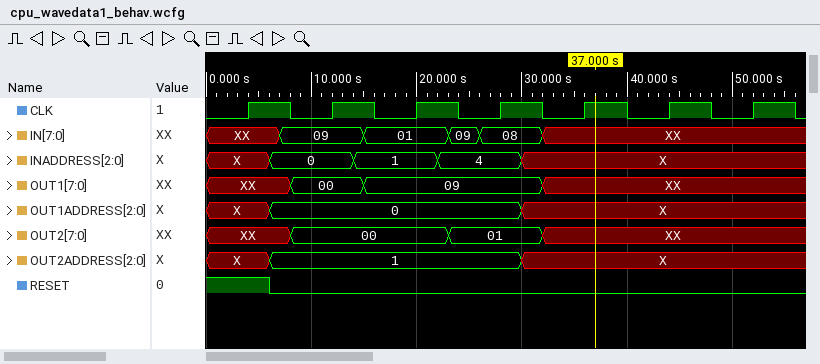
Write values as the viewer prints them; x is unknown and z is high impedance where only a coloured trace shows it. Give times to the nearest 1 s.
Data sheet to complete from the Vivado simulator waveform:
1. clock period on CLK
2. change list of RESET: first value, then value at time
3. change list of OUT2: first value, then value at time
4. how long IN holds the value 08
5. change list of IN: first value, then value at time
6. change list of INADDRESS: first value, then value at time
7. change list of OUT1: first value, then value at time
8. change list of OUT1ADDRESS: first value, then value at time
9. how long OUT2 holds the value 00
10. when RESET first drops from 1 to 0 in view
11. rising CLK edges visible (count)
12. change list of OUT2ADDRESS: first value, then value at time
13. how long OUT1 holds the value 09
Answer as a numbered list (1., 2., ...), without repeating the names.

1. 8 s
2. 1, 0 at 6 s
3. XX, 00 at 8 s, 01 at 23 s, XX at 32 s
4. 6 s
5. XX, 09 at 7 s, 01 at 15 s, 09 at 23 s, 08 at 26 s, XX at 32 s
6. X, 0 at 6 s, 1 at 14 s, 4 at 22 s, X at 30 s
7. XX, 00 at 8 s, 09 at 15 s, XX at 32 s
8. X, 0 at 6 s, X at 30 s
9. 15 s
10. 6 s
11. 7
12. X, 1 at 6 s, X at 30 s
13. 17 s
